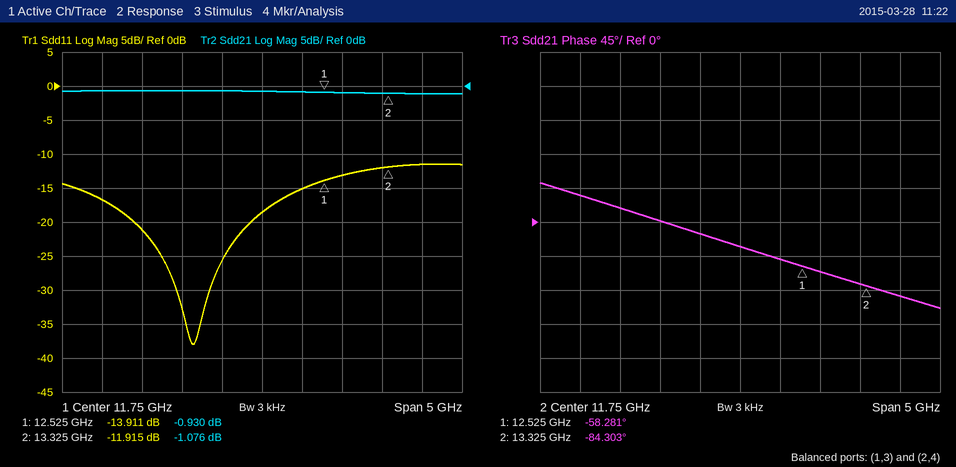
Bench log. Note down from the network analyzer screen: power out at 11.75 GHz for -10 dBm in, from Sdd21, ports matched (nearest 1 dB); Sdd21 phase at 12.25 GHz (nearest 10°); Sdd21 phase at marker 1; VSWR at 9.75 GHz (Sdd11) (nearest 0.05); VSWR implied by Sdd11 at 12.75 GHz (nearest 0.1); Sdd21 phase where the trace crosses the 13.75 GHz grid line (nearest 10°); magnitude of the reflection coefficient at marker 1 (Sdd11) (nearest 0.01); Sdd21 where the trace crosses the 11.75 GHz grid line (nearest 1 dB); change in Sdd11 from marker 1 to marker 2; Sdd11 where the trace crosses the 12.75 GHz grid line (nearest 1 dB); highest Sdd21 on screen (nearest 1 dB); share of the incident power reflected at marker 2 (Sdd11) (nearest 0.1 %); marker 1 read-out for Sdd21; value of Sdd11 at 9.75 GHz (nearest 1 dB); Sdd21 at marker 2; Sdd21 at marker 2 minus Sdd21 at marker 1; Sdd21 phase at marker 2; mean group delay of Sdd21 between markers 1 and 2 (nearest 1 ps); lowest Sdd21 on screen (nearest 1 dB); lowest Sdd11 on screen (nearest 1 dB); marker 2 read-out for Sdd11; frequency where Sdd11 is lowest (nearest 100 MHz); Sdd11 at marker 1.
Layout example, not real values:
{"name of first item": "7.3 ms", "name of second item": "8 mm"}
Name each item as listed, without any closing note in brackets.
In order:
{"power out at 11.75 GHz for -10 dBm in, from Sdd21, ports matched": "-11 dBm", "Sdd21 phase at 12.25 GHz": "-50°", "Sdd21 phase at marker 1": "-58.281°", "VSWR at 9.75 GHz (Sdd11)": "1.35", "VSWR implied by Sdd11 at 12.75 GHz": "1.6", "Sdd21 phase where the trace crosses the 13.75 GHz grid line": "-100°", "magnitude of the reflection coefficient at marker 1 (Sdd11)": "0.20", "Sdd21 where the trace crosses the 11.75 GHz grid line": "-1 dB", "change in Sdd11 from marker 1 to marker 2": "1.996 dB", "Sdd11 where the trace crosses the 12.75 GHz grid line": "-13 dB", "highest Sdd21 on screen": "-1 dB", "share of the incident power reflected at marker 2 (Sdd11)": "6.4 %", "marker 1 read-out for Sdd21": "-0.930 dB", "value of Sdd11 at 9.75 GHz": "-17 dB", "Sdd21 at marker 2": "-1.076 dB", "Sdd21 at marker 2 minus Sdd21 at marker 1": "-0.146 dB", "Sdd21 phase at marker 2": "-84.303°", "mean group delay of Sdd21 between markers 1 and 2": "90 ps", "lowest Sdd21 on screen": "-1 dB", "lowest Sdd11 on screen": "-38 dB", "marker 2 read-out for Sdd11": "-11.915 dB", "frequency where Sdd11 is lowest": "10.9 GHz", "Sdd11 at marker 1": "-13.911 dB"}
